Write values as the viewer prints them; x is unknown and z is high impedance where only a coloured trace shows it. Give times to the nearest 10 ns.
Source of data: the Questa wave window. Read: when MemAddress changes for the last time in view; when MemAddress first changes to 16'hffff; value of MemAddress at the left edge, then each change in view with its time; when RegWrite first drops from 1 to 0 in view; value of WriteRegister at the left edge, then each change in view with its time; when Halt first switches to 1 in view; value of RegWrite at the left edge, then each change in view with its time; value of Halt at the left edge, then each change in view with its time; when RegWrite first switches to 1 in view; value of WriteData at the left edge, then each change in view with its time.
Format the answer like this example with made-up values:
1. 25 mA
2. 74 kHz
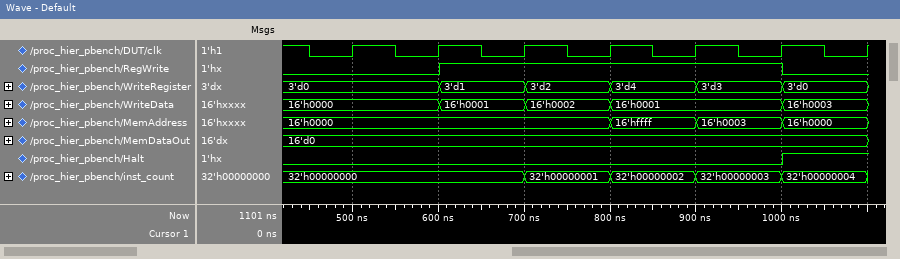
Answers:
1. 1000 ns
2. 800 ns
3. 16'h0000, 16'hffff at 800 ns, 16'h0003 at 900 ns, 16'h0000 at 1000 ns
4. 1000 ns
5. 3'd0, 3'd1 at 600 ns, 3'd2 at 700 ns, 3'd4 at 800 ns, 3'd3 at 900 ns, 3'd0 at 1000 ns
6. 1000 ns
7. 0, 1 at 600 ns, 0 at 1000 ns
8. 0, 1 at 1000 ns
9. 600 ns
10. 16'h0000, 16'h0001 at 600 ns, 16'h0002 at 700 ns, 16'h0001 at 800 ns, 16'h0003 at 1000 ns
